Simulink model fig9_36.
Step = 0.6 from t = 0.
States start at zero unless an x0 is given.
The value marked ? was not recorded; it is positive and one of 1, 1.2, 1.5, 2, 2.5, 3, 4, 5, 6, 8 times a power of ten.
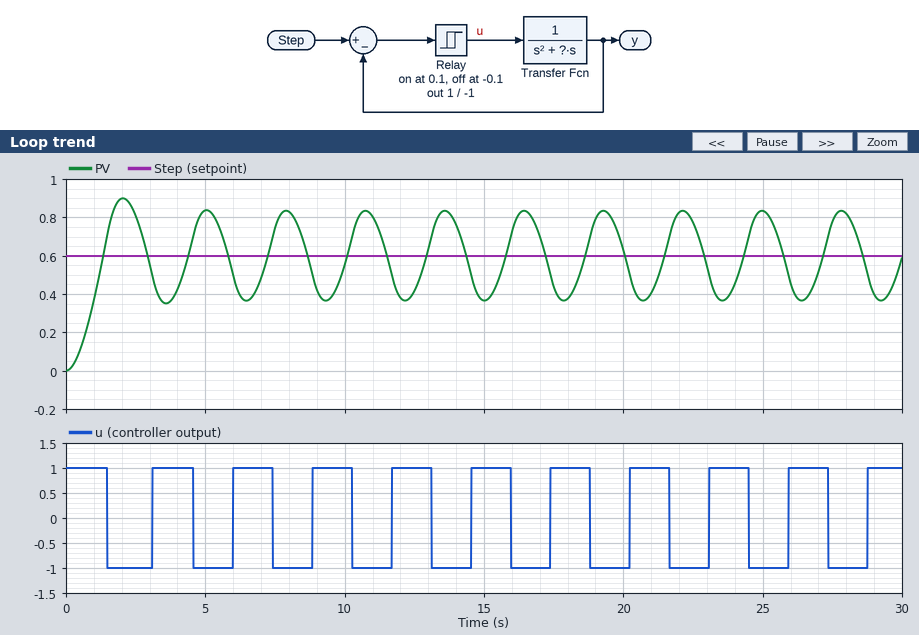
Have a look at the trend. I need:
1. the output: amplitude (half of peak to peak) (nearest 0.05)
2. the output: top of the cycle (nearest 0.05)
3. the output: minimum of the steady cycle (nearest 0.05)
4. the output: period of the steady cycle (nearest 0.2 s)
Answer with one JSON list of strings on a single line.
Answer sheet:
["0.25", "0.85", "0.35", "2.8 s"]
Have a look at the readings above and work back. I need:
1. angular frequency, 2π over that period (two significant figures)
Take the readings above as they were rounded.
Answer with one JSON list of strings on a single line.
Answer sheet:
["2.2 rad/s"]
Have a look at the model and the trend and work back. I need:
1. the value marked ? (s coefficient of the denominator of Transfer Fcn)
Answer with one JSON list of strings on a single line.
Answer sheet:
["1"]
